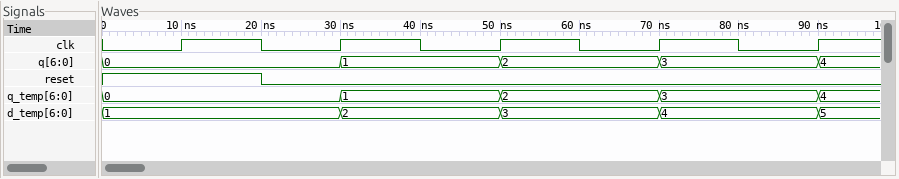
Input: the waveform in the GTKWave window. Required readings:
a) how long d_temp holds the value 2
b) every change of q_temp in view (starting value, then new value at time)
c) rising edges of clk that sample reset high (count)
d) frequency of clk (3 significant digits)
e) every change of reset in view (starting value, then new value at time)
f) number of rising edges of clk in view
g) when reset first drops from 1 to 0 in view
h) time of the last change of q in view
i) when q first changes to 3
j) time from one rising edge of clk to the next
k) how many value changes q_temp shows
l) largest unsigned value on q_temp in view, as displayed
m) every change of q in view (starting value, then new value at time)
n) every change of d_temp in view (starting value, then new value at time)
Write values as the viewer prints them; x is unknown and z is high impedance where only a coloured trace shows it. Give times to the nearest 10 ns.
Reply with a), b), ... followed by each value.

a) 20 ns
b) 0, 1 at 30 ns, 2 at 50 ns, 3 at 70 ns, 4 at 90 ns
c) 1
d) 50.0 MHz
e) 1, 0 at 20 ns
f) 5
g) 20 ns
h) 90 ns
i) 70 ns
j) 20 ns
k) 4
l) 4
m) 0, 1 at 30 ns, 2 at 50 ns, 3 at 70 ns, 4 at 90 ns
n) 1, 2 at 30 ns, 3 at 50 ns, 4 at 70 ns, 5 at 90 ns
